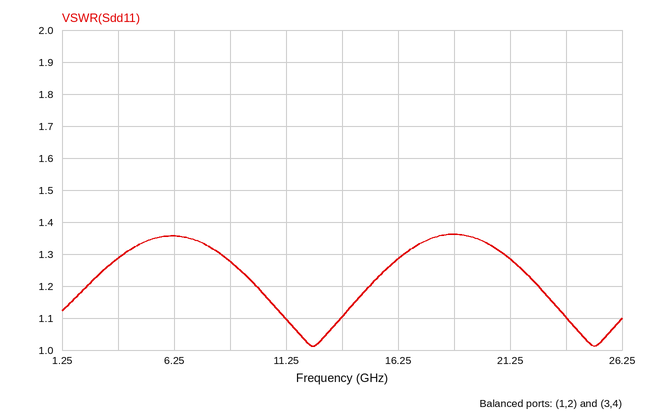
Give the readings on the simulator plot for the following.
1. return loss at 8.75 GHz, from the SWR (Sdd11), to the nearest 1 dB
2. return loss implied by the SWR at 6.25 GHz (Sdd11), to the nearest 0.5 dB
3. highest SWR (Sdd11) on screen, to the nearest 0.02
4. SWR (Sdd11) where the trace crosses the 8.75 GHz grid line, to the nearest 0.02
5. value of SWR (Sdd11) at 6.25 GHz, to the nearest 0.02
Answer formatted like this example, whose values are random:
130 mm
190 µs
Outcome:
18 dB
16.5 dB
1.36
1.28
1.36
